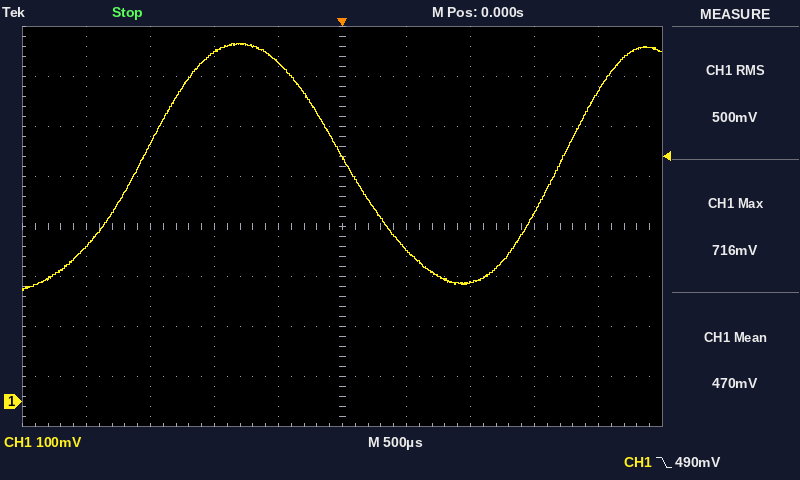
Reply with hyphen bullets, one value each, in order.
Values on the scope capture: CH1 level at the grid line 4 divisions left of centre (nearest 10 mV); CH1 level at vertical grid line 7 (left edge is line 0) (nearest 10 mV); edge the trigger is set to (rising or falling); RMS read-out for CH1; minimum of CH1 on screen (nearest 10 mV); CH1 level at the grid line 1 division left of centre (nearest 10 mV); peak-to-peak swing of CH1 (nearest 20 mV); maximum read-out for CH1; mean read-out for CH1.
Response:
- 310 mV
- 240 mV
- falling
- 500 mV
- 220 mV
- 680 mV
- 500 mV
- 716 mV
- 470 mV
